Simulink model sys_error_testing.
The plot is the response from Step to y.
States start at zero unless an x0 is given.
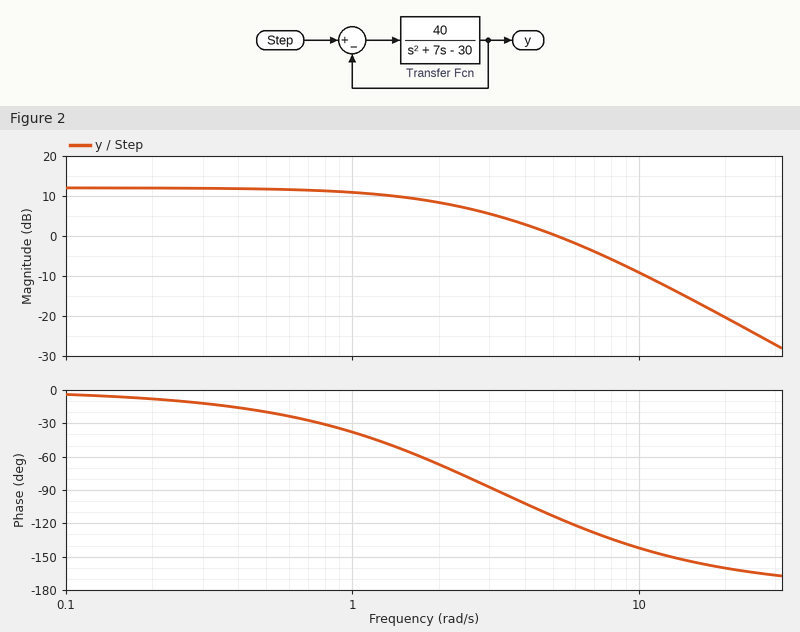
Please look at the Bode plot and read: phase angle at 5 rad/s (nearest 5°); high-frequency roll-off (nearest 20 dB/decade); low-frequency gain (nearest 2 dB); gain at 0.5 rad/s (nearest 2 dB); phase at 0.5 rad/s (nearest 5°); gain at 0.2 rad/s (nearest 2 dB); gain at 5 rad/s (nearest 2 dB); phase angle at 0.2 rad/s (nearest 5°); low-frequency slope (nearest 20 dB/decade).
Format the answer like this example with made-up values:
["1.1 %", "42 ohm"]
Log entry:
["-115°", "-40 dB/decade", "12 dB", "12 dB", "-20°", "12 dB", "0 dB", "-10°", "0 dB/decade"]
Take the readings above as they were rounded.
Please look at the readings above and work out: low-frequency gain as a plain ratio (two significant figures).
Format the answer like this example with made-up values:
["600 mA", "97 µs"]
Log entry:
["4.0"]
